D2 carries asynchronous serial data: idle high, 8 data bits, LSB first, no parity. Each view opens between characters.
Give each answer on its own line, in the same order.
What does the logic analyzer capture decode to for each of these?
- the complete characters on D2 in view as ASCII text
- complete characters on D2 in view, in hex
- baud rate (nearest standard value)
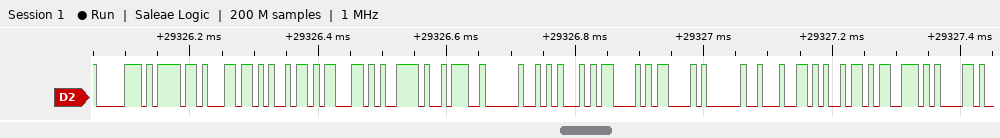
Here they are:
"policy: ECC disa"
70, 6F, 6C, 69, 63, 79, 3A, 20, 45, 43, 43, 20, 64, 69, 73, 61
115200 baud
